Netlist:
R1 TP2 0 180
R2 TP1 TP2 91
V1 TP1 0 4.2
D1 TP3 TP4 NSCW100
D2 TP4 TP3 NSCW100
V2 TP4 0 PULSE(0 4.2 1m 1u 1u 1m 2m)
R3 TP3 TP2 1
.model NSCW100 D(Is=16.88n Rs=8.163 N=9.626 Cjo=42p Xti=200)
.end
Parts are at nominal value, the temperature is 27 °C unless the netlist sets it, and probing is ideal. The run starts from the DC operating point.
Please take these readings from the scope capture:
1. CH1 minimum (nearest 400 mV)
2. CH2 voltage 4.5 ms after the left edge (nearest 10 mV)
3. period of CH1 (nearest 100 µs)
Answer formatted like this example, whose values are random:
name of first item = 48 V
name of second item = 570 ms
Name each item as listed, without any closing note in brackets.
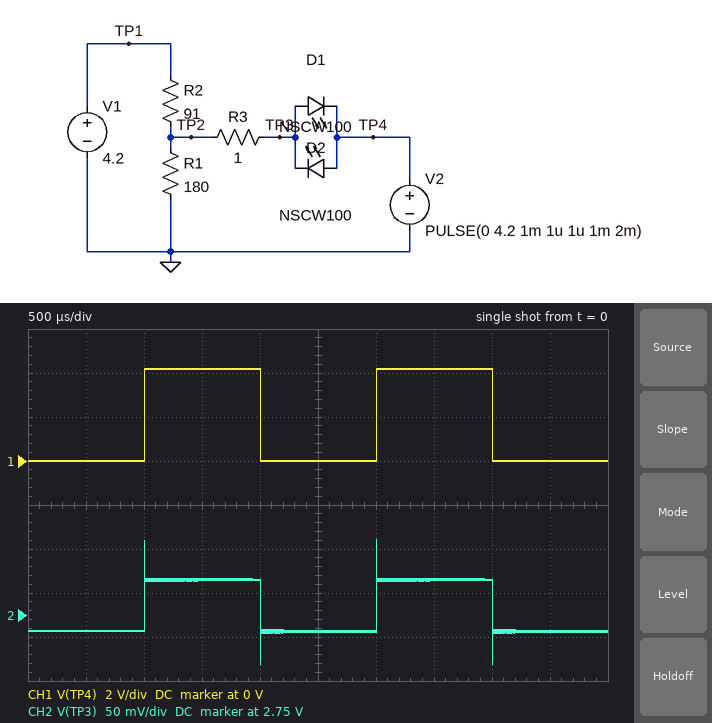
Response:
CH1 minimum = 0 V
CH2 voltage 4.5 ms after the left edge = 2.73 V
period of CH1 = 2.0 ms
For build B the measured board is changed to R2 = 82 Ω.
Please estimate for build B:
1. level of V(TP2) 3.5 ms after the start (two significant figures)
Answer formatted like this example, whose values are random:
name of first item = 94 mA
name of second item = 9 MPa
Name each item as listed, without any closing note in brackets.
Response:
level of V(TP2) 3.5 ms after the start = 2.9 V
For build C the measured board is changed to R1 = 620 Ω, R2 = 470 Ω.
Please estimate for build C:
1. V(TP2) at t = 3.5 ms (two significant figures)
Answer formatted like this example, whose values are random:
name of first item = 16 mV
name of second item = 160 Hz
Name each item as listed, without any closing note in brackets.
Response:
V(TP2) at t = 3.5 ms = 2.4 V
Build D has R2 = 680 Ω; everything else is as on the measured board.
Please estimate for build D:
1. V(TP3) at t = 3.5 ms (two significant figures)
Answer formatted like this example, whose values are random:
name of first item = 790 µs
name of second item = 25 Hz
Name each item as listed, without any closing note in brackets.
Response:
V(TP3) at t = 3.5 ms = 1.2 V
